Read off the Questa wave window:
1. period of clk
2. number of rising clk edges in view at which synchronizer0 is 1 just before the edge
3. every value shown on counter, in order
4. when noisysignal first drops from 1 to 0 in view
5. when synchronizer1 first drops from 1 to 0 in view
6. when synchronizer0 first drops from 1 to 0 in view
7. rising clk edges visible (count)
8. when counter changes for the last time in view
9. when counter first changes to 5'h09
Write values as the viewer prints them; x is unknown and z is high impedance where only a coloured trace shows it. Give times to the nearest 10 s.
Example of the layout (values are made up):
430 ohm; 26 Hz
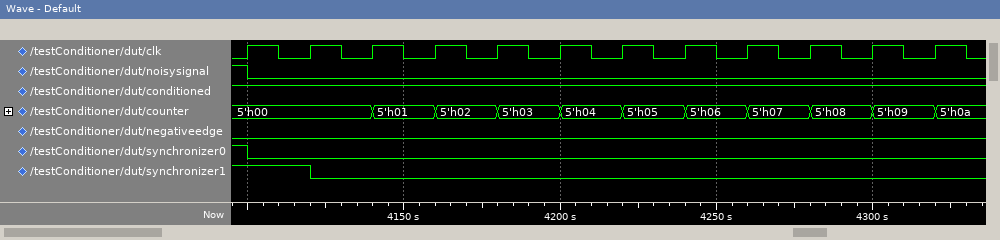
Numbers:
20 s; 1; 5'h00, 5'h01, 5'h02, 5'h03, 5'h04, 5'h05, 5'h06, 5'h07, 5'h08, 5'h09, 5'h0a; 4100 s; 4120 s; 4100 s; 12; 4320 s; 4300 s
